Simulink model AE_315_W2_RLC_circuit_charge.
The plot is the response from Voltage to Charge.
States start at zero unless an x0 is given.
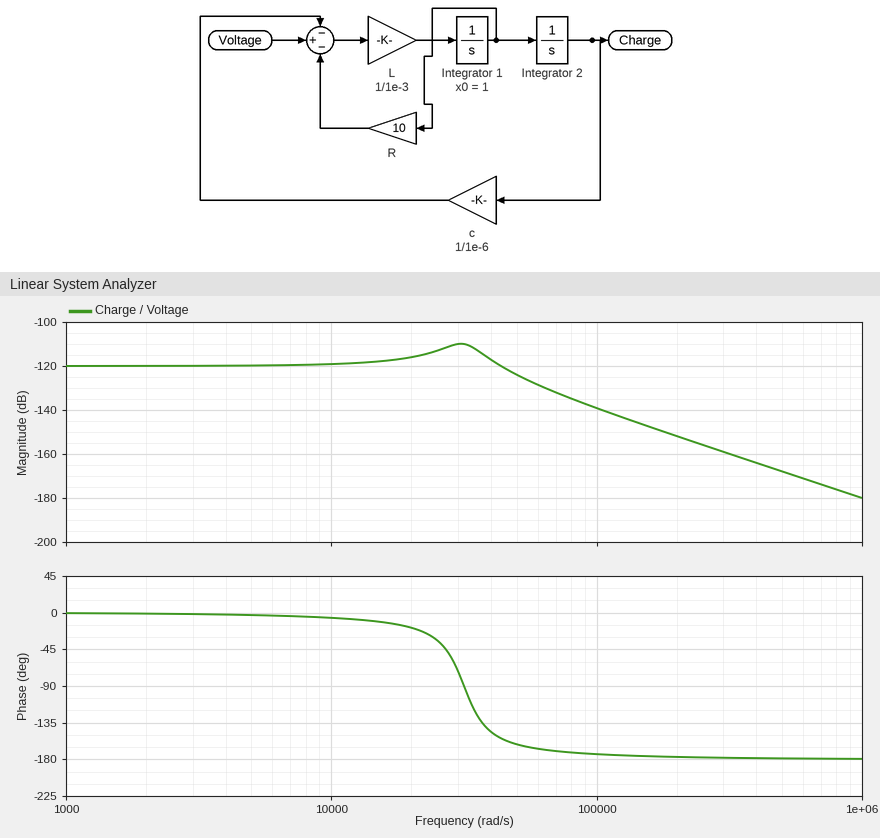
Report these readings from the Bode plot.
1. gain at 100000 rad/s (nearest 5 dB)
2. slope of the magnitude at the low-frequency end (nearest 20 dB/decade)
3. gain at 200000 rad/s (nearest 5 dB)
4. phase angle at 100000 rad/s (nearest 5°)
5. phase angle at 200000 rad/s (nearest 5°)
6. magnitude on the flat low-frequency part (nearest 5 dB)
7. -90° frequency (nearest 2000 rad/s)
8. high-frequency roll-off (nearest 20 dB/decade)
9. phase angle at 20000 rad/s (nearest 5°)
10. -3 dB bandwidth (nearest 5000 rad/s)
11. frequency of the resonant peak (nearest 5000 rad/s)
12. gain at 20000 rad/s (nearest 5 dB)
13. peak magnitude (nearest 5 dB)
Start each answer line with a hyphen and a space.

- -140 dB
- 0 dB/decade
- -150 dB
- -175°
- -175°
- -120 dB
- 32000 rad/s
- -40 dB/decade
- -20°
- 50000 rad/s
- 30000 rad/s
- -115 dB
- -110 dB
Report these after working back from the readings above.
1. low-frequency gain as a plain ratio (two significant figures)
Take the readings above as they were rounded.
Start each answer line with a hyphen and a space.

- 0.0000010
